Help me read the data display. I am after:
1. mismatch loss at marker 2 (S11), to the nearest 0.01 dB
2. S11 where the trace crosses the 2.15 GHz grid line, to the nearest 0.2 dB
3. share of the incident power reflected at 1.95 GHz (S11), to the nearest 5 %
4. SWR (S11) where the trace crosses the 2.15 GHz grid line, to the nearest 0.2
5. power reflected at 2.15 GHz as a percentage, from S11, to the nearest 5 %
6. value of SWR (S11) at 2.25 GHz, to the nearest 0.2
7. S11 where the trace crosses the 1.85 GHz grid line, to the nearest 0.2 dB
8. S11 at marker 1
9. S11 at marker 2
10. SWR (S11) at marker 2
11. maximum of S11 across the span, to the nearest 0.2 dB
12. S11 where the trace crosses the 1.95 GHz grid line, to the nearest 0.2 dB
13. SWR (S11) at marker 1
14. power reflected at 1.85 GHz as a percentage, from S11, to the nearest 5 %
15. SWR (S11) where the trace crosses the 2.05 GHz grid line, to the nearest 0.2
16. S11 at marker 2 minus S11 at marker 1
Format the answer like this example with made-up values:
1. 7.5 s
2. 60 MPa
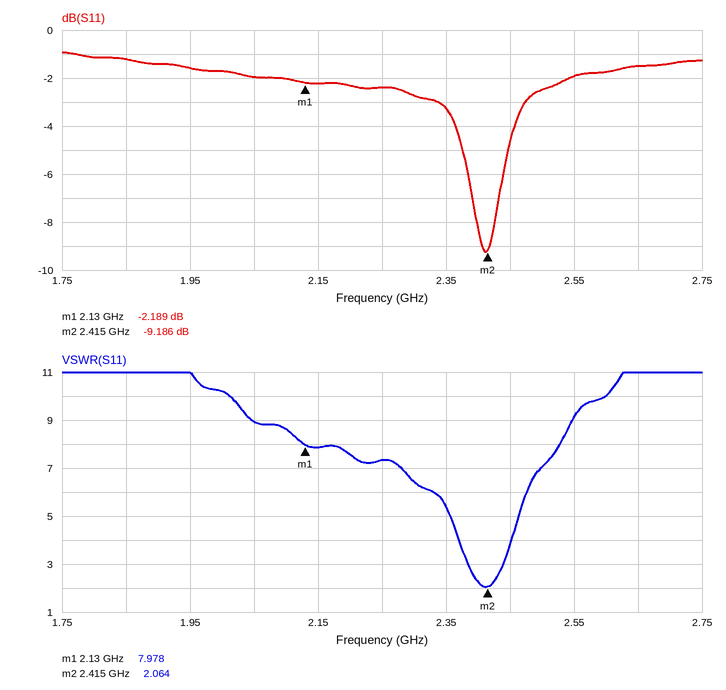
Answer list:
1. 0.56 dB
2. -2.2 dB
3. 70 %
4. 7.8
5. 60 %
6. 7.4
7. -1.2 dB
8. -2.189 dB
9. -9.186 dB
10. 2.064
11. -1.0 dB
12. -1.6 dB
13. 7.978
14. 75 %
15. 9.0
16. -6.997 dB
